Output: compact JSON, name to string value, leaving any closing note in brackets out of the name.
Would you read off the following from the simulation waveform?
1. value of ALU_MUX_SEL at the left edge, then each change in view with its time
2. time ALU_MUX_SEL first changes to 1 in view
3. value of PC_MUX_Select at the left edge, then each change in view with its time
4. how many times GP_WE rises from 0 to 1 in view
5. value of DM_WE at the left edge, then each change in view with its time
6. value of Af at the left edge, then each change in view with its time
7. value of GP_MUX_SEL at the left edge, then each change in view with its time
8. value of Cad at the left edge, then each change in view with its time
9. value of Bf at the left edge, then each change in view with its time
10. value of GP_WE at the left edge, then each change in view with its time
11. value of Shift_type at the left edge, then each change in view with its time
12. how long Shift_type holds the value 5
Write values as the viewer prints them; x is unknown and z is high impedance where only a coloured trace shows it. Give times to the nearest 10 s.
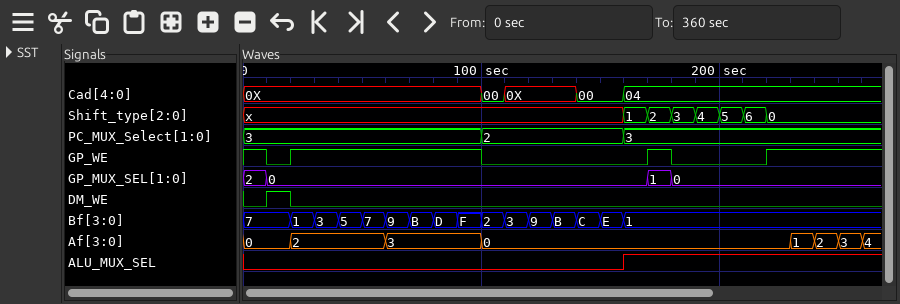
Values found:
{"value of ALU_MUX_SEL at the left edge, then each change in view with its time": "0, 1 at 160 s", "time ALU_MUX_SEL first changes to 1 in view": "160 s", "value of PC_MUX_Select at the left edge, then each change in view with its time": "3, 2 at 100 s, 3 at 160 s", "how many times GP_WE rises from 0 to 1 in view": "3", "value of DM_WE at the left edge, then each change in view with its time": "0, 1 at 10 s, 0 at 20 s", "value of Af at the left edge, then each change in view with its time": "0, 2 at 20 s, 3 at 60 s, 0 at 100 s, 1 at 230 s, 2 at 240 s, 3 at 250 s, 4 at 260 s", "value of GP_MUX_SEL at the left edge, then each change in view with its time": "2, 0 at 10 s, 1 at 170 s, 0 at 180 s", "value of Cad at the left edge, then each change in view with its time": "0X, 00 at 100 s, 0X at 110 s, 00 at 140 s, 04 at 160 s", "value of Bf at the left edge, then each change in view with its time": "7, 1 at 20 s, 3 at 30 s, 5 at 40 s, 7 at 50 s, 9 at 60 s, B at 70 s, D at 80 s, F at 90 s, 2 at 100 s, 3 at 110 s, 9 at 120 s, B at 130 s, C at 140 s, E at 150 s, 1 at 160 s", "value of GP_WE at the left edge, then each change in view with its time": "1, 0 at 10 s, 1 at 20 s, 0 at 100 s, 1 at 170 s, 0 at 180 s, 1 at 220 s", "value of Shift_type at the left edge, then each change in view with its time": "x, 1 at 160 s, 2 at 170 s, 3 at 180 s, 4 at 190 s, 5 at 200 s, 6 at 210 s, 0 at 220 s", "how long Shift_type holds the value 5": "10 s"}
